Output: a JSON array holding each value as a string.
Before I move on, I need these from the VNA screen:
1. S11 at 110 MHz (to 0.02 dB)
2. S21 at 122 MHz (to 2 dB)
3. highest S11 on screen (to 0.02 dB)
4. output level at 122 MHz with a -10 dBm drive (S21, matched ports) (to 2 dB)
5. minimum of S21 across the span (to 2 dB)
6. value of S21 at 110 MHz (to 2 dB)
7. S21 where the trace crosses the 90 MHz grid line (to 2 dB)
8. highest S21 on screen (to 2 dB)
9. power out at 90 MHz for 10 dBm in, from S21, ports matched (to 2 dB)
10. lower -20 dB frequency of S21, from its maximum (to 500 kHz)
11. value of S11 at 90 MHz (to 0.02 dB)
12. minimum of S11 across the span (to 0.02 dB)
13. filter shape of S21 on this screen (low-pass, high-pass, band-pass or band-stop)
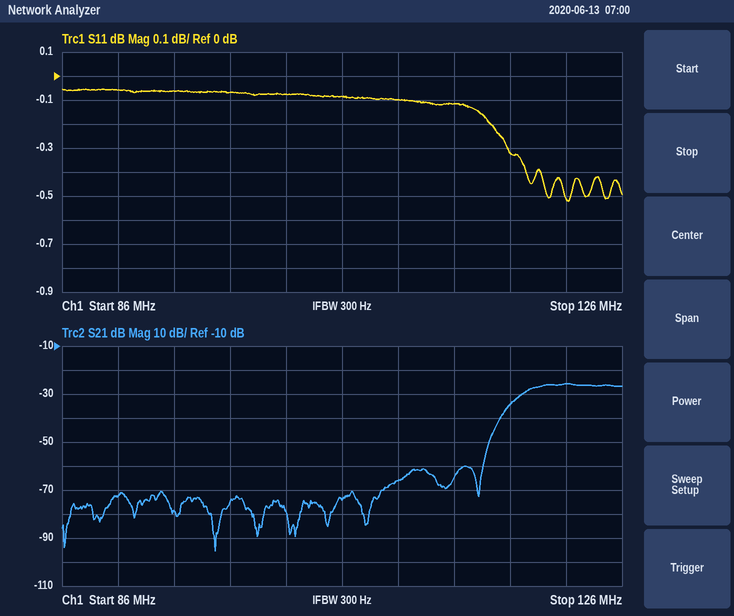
["-0.10 dB", "-26 dB", "-0.06 dB", "-36 dBm", "-96 dB", "-66 dB", "-72 dB", "-26 dB", "-62 dBm", "117.0 MHz", "-0.06 dB", "-0.52 dB", "high-pass"]
